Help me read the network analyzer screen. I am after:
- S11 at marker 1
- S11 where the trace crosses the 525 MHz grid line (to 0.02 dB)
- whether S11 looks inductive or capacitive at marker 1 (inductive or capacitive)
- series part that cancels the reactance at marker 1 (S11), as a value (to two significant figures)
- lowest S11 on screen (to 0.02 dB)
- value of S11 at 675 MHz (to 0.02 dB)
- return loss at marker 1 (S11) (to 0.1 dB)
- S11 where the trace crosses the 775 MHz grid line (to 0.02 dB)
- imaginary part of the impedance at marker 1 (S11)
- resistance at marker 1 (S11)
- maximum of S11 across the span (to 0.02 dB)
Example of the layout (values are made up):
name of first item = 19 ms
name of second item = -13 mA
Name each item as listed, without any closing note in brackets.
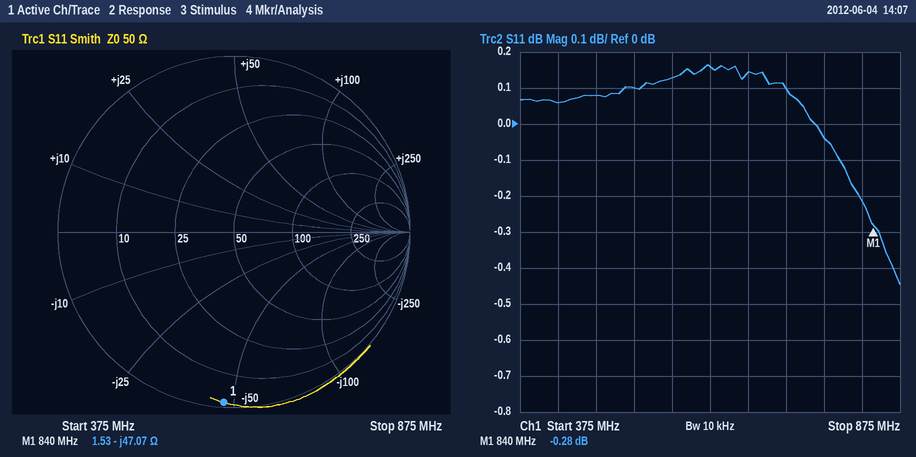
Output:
S11 at marker 1 = -0.28 dB
S11 where the trace crosses the 525 MHz grid line = 0.10 dB
whether S11 looks inductive or capacitive at marker 1 = capacitive
series part that cancels the reactance at marker 1 (S11), as a value = 8.9 nH
lowest S11 on screen = -0.44 dB
value of S11 at 675 MHz = 0.14 dB
return loss at marker 1 (S11) = 0.3 dB
S11 where the trace crosses the 775 MHz grid line = -0.04 dB
imaginary part of the impedance at marker 1 = -47.07 Ω
resistance at marker 1 = 1.53 Ω
maximum of S11 across the span = 0.16 dB
